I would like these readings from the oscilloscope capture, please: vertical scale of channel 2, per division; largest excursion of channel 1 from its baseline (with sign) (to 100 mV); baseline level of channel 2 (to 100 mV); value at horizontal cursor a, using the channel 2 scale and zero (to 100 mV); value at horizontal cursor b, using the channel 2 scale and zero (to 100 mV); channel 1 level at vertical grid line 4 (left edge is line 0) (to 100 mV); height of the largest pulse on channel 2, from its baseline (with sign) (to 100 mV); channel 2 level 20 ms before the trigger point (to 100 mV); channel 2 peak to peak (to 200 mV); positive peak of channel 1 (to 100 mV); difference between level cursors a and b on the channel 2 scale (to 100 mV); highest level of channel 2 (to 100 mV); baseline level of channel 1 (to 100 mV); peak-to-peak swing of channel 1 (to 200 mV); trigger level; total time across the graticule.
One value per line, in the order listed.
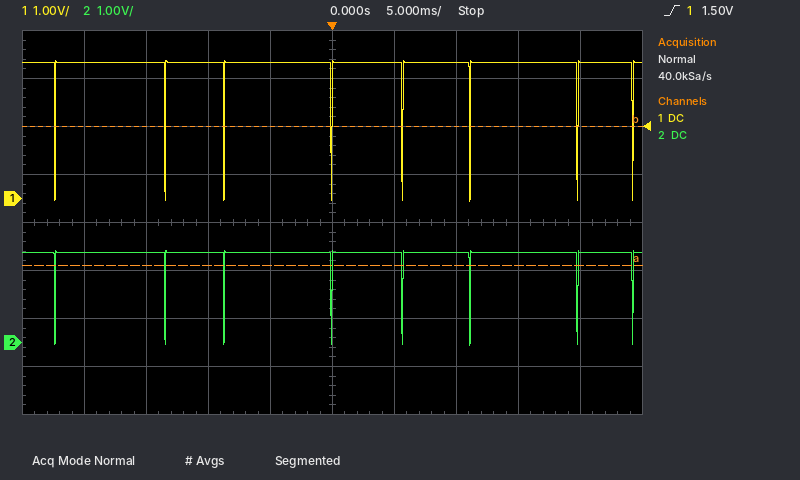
1 V
-2.9 V
1.9 V
1.6 V
4.5 V
2.8 V
-1.9 V
1.9 V
2.0 V
2.9 V
2.9 V
1.9 V
2.8 V
3.0 V
1.50 V
50 ms
